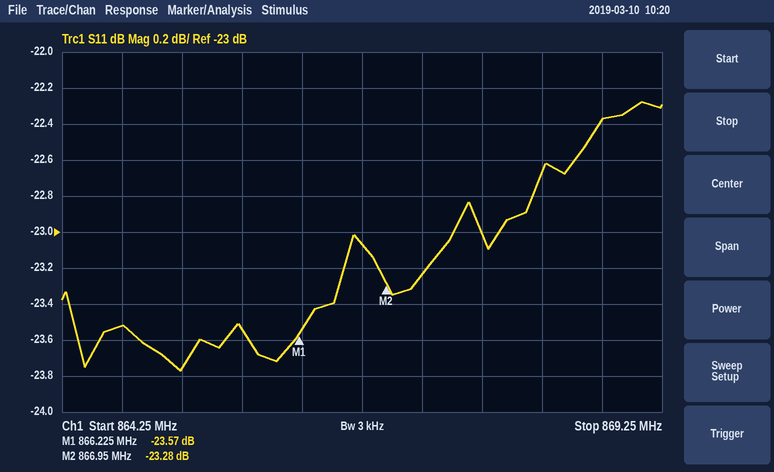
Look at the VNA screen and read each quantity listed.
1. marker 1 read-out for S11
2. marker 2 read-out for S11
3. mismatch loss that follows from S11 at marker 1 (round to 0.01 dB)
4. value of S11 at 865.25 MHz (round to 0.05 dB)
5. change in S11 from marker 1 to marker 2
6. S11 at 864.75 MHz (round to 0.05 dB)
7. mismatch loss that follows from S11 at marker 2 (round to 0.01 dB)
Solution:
-23.57 dB
-23.28 dB
0.02 dB
-23.75 dB
0.29 dB
-23.50 dB
0.02 dB
